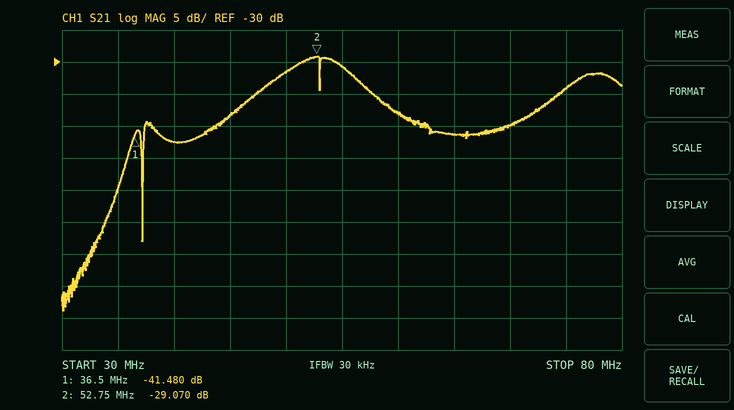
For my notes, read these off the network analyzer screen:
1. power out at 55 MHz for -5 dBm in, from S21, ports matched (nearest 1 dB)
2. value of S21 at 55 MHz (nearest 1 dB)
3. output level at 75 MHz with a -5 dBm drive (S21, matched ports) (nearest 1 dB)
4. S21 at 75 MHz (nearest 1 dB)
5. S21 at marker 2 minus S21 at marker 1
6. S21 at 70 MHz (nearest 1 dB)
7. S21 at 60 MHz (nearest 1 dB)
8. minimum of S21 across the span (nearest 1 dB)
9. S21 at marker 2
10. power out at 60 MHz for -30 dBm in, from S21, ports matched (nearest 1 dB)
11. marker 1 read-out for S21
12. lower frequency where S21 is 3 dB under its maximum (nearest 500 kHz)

-36 dBm
-31 dB
-39 dBm
-34 dB
12.410 dB
-40 dB
-38 dB
-69 dB
-29.070 dB
-68 dBm
-41.480 dB
49.5 MHz
